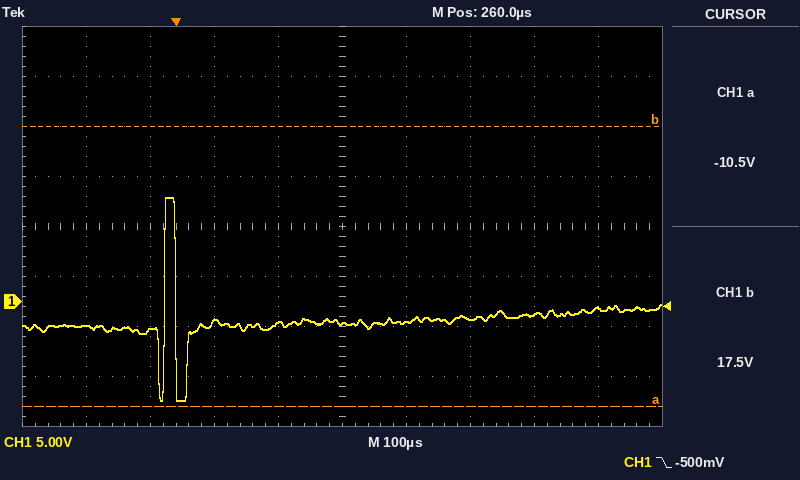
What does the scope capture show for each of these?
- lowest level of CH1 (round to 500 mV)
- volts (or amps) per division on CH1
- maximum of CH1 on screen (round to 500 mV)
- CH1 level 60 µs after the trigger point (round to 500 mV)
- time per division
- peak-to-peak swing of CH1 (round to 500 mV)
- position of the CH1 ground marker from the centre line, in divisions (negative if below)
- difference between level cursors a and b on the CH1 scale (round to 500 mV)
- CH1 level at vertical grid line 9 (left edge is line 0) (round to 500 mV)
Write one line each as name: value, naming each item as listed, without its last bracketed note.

lowest level of CH1: -10.0 V
volts (or amps) per division on CH1: 5 V
maximum of CH1 on screen: 10.5 V
CH1 level 60 µs after the trigger point: -2.0 V
time per division: 100 µs
peak-to-peak swing of CH1: 20.5 V
position of the CH1 ground marker from the centre line, in divisions: -1.5 div
difference between level cursors a and b on the CH1 scale: 28.0 V
CH1 level at vertical grid line 9 (left edge is line 0): -500 mV
